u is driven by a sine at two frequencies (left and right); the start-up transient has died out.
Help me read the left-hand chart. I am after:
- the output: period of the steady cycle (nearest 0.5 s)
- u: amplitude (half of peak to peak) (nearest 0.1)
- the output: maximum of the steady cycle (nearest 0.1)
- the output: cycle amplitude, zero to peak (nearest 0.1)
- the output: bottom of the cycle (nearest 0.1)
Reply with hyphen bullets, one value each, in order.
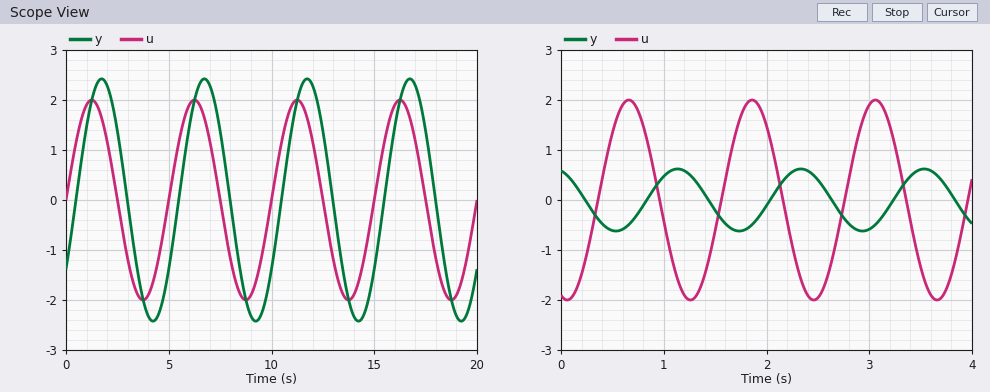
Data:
- 5.0 s
- 2.0
- 2.4
- 2.4
- -2.4
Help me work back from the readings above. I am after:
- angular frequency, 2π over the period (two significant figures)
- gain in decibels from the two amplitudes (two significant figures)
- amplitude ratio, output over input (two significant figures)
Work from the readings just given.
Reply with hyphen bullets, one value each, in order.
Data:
- 1.3 rad/s
- 1.6 dB
- 1.2
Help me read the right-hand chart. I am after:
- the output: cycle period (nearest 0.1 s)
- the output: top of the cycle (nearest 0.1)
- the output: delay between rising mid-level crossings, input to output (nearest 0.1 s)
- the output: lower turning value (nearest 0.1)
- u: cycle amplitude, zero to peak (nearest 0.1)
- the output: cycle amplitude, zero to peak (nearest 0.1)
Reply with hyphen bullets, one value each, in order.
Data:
- 1.2 s
- 0.6
- 0.5 s
- -0.6
- 2.0
- 0.6
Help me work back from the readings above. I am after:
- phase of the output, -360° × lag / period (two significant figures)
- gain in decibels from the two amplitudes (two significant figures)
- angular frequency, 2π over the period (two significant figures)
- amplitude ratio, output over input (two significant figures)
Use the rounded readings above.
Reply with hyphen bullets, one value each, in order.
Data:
- -150°
- -10 dB
- 5.2 rad/s
- 0.30
